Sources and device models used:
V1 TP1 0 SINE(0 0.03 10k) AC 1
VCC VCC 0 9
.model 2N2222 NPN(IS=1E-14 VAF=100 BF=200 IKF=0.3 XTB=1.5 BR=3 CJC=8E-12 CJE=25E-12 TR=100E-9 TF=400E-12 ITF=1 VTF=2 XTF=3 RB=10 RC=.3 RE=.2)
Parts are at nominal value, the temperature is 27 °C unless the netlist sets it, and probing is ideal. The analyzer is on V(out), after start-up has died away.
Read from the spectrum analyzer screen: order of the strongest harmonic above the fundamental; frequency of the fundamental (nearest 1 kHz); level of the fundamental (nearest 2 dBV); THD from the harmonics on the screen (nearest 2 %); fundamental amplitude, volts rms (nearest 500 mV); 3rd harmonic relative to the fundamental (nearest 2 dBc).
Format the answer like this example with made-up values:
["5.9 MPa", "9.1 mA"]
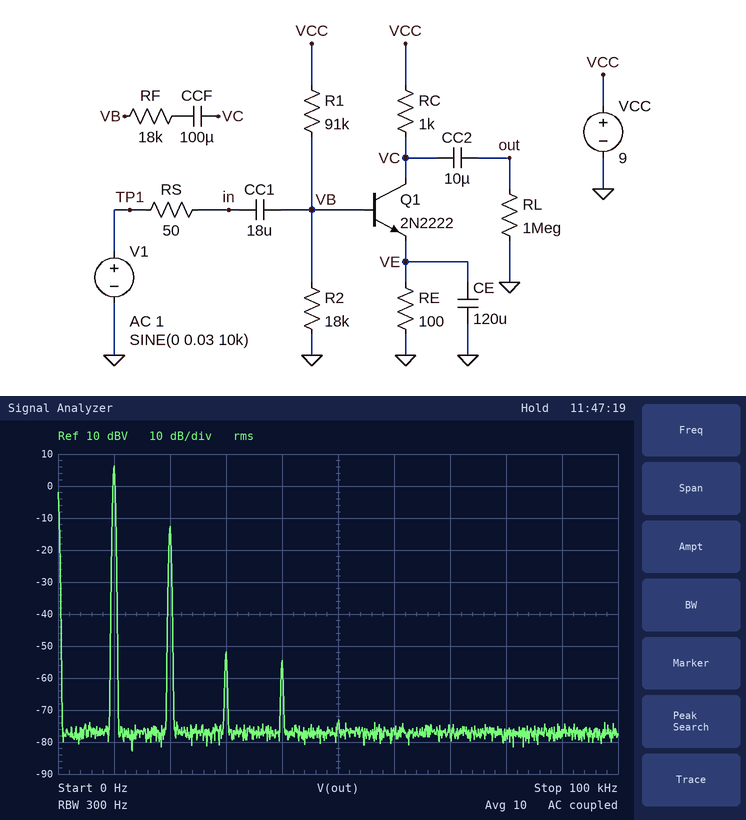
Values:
["2", "10 kHz", "6 dBV", "12 %", "2.0 V", "-58 dBc"]
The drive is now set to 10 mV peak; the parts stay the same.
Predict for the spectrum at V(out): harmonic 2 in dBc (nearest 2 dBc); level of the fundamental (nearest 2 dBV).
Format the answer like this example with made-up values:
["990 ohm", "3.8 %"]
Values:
["-28 dBc", "-2 dBV"]
